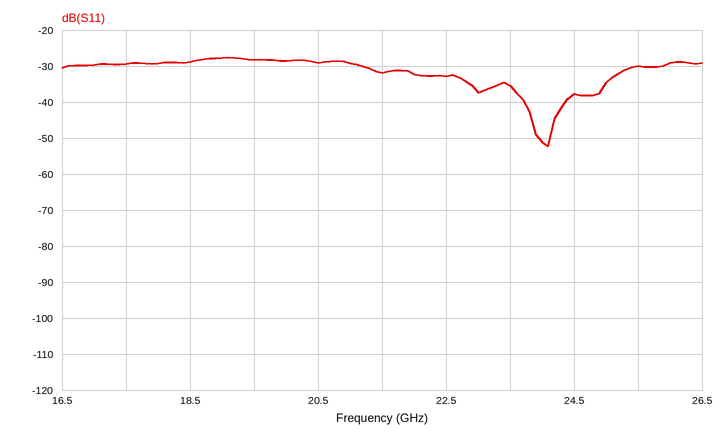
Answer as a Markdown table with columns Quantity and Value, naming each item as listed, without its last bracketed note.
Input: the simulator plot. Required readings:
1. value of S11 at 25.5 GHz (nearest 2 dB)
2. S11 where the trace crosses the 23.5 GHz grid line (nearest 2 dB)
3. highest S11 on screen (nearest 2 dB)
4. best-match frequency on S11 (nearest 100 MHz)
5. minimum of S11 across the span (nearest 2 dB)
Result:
| Quantity | Value |
|---|---|
| value of S11 at 25.5 GHz | -30 dB |
| S11 where the trace crosses the 23.5 GHz grid line | -36 dB |
| highest S11 on screen | -28 dB |
| best-match frequency on S11 | 24.1 GHz |
| minimum of S11 across the span | -52 dB |
